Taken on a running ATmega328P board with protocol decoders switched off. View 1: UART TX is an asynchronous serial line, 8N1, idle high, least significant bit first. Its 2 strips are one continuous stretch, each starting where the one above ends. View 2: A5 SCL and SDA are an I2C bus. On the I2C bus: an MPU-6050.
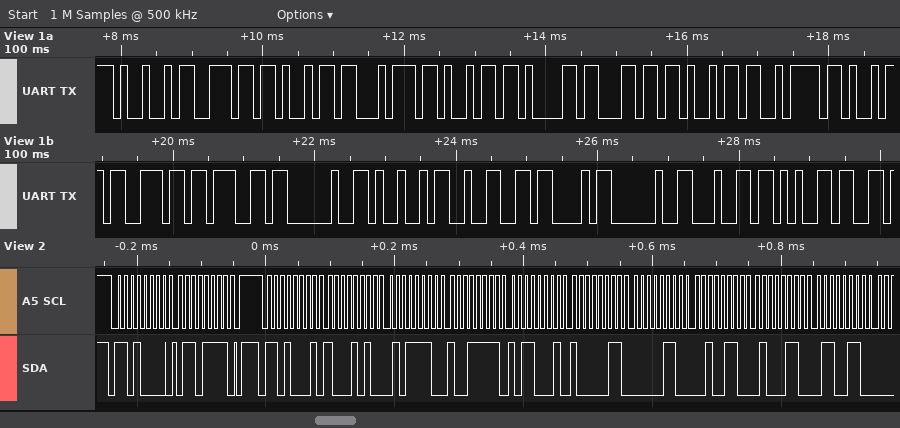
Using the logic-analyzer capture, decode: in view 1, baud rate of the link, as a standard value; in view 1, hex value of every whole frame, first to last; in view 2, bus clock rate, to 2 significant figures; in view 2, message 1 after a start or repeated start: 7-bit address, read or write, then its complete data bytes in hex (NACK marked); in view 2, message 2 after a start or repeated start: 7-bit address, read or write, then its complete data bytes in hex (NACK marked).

9600 baud
49 6E 69 74 69 61 6C 69 7A 69 6E 67 20 49 32 43 20 64 65
100 kHz
0x68 write: 6F
0x68 read: 8A 5E 9F B1 83 06 26 46 66
